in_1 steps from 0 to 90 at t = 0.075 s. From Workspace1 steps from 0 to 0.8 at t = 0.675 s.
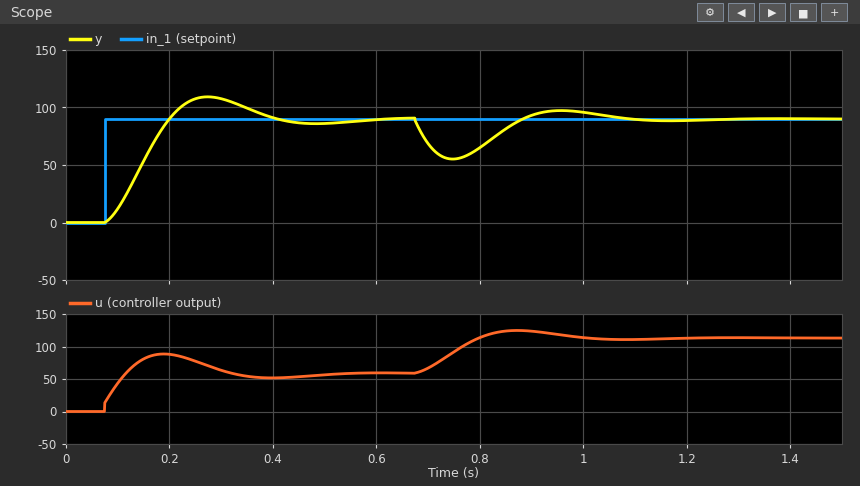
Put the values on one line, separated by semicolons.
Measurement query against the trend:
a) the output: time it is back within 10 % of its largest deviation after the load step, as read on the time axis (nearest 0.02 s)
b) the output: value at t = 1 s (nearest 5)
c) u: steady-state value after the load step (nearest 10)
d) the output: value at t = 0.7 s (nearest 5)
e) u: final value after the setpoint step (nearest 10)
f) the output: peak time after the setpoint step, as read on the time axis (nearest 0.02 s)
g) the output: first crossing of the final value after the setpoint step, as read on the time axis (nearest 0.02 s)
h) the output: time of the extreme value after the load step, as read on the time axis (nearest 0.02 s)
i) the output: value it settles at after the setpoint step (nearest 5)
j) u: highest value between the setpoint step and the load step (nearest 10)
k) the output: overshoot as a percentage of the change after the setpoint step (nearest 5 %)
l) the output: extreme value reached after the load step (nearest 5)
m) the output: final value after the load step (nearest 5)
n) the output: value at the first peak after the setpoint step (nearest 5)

1.04 s; 95; 110; 70; 60; 0.28 s; 0.20 s; 0.74 s; 90; 90; 20 %; 55; 90; 110
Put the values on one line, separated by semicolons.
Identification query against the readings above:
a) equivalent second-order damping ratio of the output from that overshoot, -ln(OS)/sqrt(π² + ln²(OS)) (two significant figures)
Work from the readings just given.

0.46
